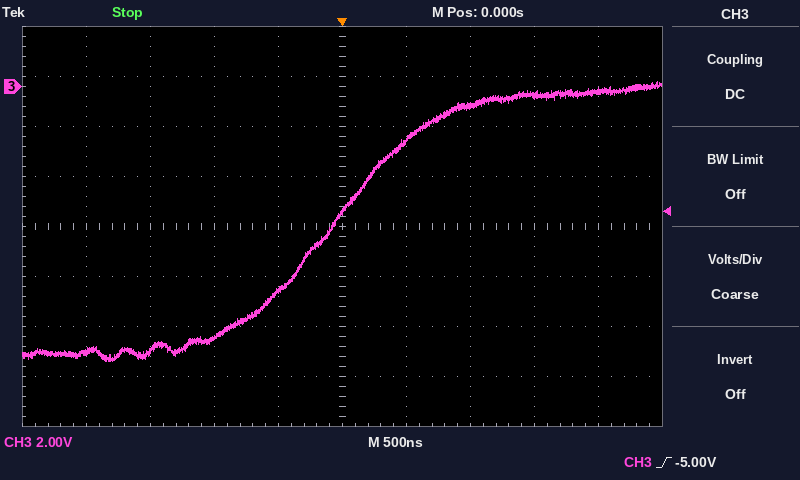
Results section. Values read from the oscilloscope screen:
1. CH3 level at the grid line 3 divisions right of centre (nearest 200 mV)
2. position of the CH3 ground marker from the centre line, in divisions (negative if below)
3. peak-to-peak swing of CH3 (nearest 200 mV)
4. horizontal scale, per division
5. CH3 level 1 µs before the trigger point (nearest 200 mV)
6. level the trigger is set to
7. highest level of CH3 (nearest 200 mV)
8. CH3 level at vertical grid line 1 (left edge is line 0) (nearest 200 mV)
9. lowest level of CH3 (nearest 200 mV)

-400 mV
+2.8 div
11.2 V
500 ns
-10.0 V
-5.00 V
200 mV
-10.6 V
-11.0 V
